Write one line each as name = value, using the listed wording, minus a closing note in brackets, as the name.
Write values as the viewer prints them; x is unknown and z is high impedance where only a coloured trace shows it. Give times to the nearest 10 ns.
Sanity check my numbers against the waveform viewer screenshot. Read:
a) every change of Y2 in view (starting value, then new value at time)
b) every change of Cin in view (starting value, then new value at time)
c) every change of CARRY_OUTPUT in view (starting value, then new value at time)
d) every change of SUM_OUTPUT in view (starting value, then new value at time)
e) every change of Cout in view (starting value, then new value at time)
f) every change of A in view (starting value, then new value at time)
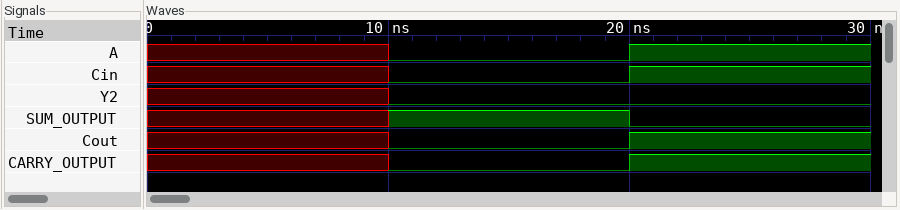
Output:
every change of Y2 in view = x, 0 at 10 ns
every change of Cin in view = x, 0 at 10 ns, 1 at 20 ns
every change of CARRY_OUTPUT in view = x, 0 at 10 ns, 1 at 20 ns
every change of SUM_OUTPUT in view = x, 1 at 10 ns, 0 at 20 ns
every change of Cout in view = x, 0 at 10 ns, 1 at 20 ns
every change of A in view = x, 0 at 10 ns, 1 at 20 ns
